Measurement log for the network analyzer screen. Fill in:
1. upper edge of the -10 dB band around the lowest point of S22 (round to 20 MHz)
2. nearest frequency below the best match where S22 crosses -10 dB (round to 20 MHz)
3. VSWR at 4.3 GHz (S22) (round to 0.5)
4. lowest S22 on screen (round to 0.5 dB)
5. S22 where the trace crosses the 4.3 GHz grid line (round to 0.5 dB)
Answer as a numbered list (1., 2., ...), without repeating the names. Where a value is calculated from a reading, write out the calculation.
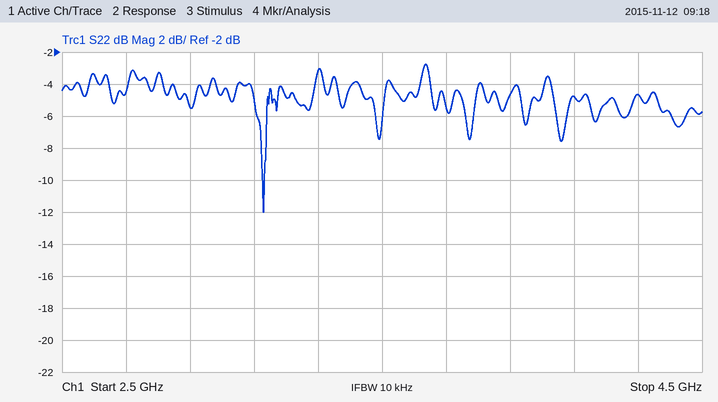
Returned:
1. 3.14 GHz
2. 3.12 GHz
3. |Γ| = 10^(-4.5/20) = 0.5957; VSWR = (1 + 0.5957)/(1 − 0.5957) ≈ 4.0
4. -12.0 dB
5. -4.5 dB
